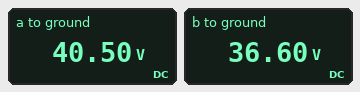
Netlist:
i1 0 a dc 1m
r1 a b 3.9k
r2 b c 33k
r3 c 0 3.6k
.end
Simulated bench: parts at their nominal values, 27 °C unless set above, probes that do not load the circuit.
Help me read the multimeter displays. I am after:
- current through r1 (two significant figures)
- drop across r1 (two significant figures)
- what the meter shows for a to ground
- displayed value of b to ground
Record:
1.0 mA
3.9 V
40.50 V
36.60 V
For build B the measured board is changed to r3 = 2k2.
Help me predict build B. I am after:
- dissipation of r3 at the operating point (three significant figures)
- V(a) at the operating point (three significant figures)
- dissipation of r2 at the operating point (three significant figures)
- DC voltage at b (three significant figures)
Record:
2.20 mW
39.1 V
33.0 mW
35.2 V
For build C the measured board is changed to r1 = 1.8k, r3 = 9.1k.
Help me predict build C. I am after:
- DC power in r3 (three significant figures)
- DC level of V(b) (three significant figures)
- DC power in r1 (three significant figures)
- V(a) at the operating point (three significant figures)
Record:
9.10 mW
42.1 V
1.80 mW
43.9 V
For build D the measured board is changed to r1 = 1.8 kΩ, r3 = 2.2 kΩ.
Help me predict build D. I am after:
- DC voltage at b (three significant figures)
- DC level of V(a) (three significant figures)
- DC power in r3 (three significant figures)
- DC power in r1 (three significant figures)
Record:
35.2 V
37.0 V
2.20 mW
1.80 mW
